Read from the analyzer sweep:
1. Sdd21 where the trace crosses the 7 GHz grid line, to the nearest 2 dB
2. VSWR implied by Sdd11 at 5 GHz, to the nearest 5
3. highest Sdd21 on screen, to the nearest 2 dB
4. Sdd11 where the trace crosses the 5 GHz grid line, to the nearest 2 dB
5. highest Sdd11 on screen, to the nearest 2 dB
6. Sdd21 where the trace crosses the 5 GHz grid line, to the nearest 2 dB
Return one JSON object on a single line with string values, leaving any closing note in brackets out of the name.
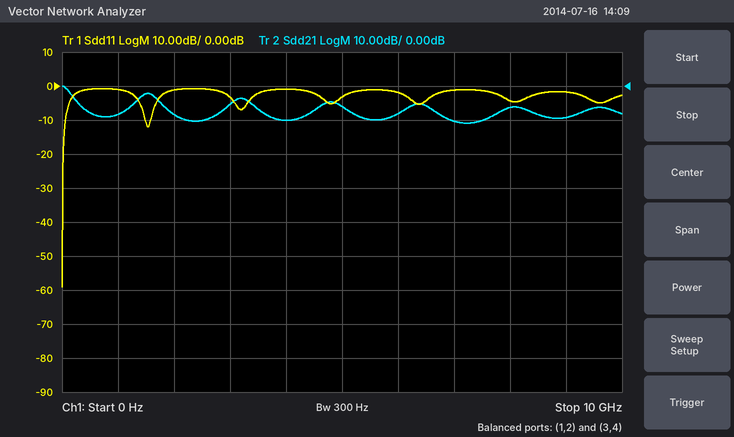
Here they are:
{"Sdd21 where the trace crosses the 7 GHz grid line, to the nearest 2 dB": "-10 dB", "VSWR implied by Sdd11 at 5 GHz, to the nearest 5": "5", "highest Sdd21 on screen, to the nearest 2 dB": "0 dB", "Sdd11 where the trace crosses the 5 GHz grid line, to the nearest 2 dB": "-4 dB", "highest Sdd11 on screen, to the nearest 2 dB": "0 dB", "Sdd21 where the trace crosses the 5 GHz grid line, to the nearest 2 dB": "-6 dB"}
